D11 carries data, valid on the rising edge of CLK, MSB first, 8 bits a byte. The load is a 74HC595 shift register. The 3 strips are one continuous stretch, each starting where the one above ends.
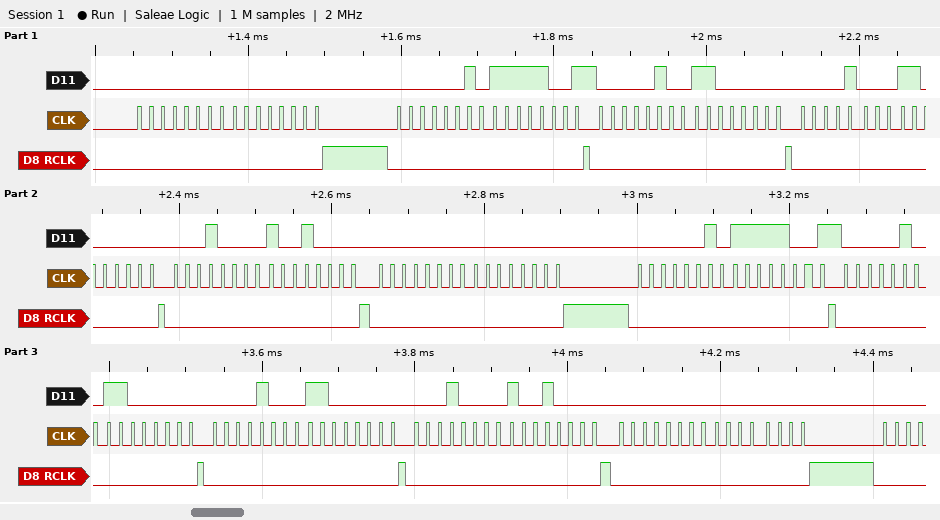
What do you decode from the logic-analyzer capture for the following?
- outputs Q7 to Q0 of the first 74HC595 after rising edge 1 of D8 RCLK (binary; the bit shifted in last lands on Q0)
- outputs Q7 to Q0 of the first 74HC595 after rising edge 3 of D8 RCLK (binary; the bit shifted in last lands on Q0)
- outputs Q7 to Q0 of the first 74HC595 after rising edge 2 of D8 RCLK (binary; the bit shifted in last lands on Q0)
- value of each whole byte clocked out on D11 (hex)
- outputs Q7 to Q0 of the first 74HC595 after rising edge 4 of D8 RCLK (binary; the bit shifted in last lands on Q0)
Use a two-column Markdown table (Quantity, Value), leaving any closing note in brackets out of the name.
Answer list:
| Quantity | Value |
|---|---|
| outputs Q7 to Q0 of the first 74HC595 after rising edge 1 of D8 RCLK | 00000000 |
| outputs Q7 to Q0 of the first 74HC595 after rising edge 3 of D8 RCLK | 11000000 |
| outputs Q7 to Q0 of the first 74HC595 after rising edge 2 of D8 RCLK | 11111001 |
| value of each whole byte clocked out on D11 | 00 00 02 F9 04 C0 08 C0 10 90 00 00 02 F9 04 C0 08 C0 10 90 00 00 |
| outputs Q7 to Q0 of the first 74HC595 after rising edge 4 of D8 RCLK | 11000000 |
